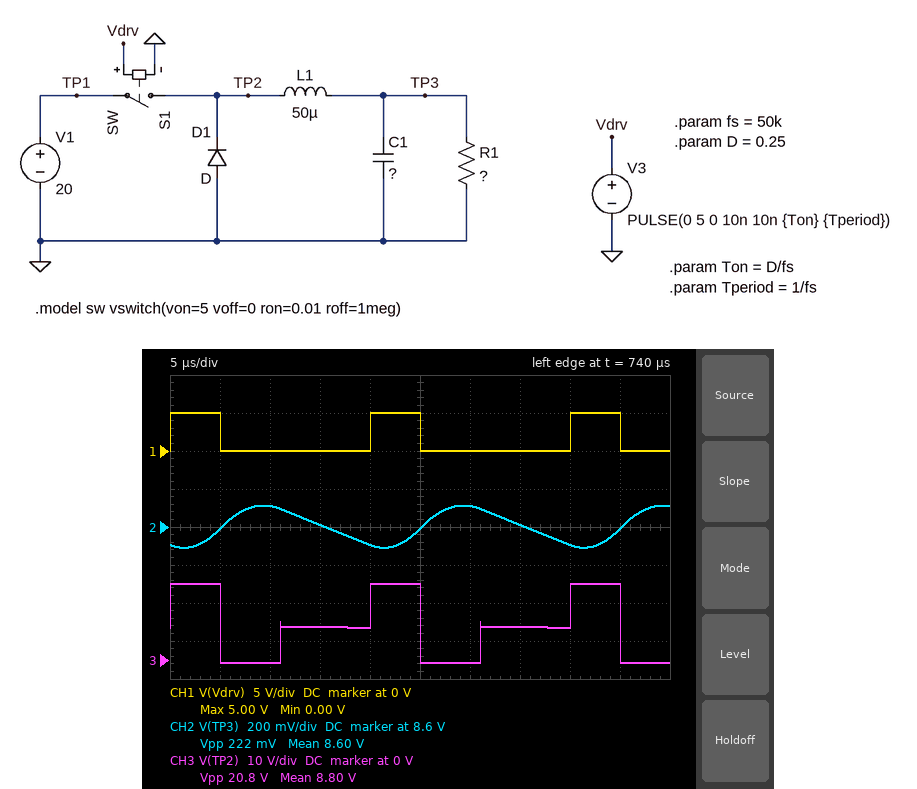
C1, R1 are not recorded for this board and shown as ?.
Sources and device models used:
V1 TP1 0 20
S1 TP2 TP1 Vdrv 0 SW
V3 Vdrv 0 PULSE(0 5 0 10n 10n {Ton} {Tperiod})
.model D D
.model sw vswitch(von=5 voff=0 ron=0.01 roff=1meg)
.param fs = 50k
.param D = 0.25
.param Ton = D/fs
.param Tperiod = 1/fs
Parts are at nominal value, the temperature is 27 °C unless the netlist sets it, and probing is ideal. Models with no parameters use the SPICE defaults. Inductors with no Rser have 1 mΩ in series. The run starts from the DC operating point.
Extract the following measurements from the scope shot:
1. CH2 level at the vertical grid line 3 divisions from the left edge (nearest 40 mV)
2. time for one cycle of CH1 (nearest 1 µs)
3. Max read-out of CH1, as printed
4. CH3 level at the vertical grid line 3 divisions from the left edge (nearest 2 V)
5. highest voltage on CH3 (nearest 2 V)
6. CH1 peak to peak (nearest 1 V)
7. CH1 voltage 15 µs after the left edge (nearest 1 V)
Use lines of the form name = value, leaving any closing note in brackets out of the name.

CH2 level at the vertical grid line 3 divisions from the left edge = 8.60 V
time for one cycle of CH1 = 20 µs
Max read-out of CH1, as printed = 5.00 V
CH3 level at the vertical grid line 3 divisions from the left edge = 8 V
highest voltage on CH3 = 20 V
CH1 peak to peak = 5 V
CH1 voltage 15 µs after the left edge = 0 V
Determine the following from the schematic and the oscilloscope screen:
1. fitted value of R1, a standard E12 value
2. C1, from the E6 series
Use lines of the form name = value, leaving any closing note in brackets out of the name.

fitted value of R1, a standard E12 value = 27 Ω
C1, from the E6 series = 15 µF
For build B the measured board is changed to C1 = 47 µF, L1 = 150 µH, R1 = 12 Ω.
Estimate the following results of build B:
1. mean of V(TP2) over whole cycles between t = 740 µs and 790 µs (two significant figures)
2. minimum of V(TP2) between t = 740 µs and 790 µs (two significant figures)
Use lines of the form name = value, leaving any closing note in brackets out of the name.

mean of V(TP2) over whole cycles between t = 740 µs and 790 µs = 4.6 V
minimum of V(TP2) between t = 740 µs and 790 µs = -820 mV
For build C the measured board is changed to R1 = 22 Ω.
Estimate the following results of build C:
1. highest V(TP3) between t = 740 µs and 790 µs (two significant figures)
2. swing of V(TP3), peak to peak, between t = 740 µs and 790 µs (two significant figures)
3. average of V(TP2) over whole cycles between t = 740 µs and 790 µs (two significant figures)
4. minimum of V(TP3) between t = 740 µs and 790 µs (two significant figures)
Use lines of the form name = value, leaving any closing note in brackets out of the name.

highest V(TP3) between t = 740 µs and 790 µs = 8.1 V
swing of V(TP3), peak to peak, between t = 740 µs and 790 µs = 240 mV
average of V(TP2) over whole cycles between t = 740 µs and 790 µs = 8.0 V
minimum of V(TP3) between t = 740 µs and 790 µs = 7.8 V
